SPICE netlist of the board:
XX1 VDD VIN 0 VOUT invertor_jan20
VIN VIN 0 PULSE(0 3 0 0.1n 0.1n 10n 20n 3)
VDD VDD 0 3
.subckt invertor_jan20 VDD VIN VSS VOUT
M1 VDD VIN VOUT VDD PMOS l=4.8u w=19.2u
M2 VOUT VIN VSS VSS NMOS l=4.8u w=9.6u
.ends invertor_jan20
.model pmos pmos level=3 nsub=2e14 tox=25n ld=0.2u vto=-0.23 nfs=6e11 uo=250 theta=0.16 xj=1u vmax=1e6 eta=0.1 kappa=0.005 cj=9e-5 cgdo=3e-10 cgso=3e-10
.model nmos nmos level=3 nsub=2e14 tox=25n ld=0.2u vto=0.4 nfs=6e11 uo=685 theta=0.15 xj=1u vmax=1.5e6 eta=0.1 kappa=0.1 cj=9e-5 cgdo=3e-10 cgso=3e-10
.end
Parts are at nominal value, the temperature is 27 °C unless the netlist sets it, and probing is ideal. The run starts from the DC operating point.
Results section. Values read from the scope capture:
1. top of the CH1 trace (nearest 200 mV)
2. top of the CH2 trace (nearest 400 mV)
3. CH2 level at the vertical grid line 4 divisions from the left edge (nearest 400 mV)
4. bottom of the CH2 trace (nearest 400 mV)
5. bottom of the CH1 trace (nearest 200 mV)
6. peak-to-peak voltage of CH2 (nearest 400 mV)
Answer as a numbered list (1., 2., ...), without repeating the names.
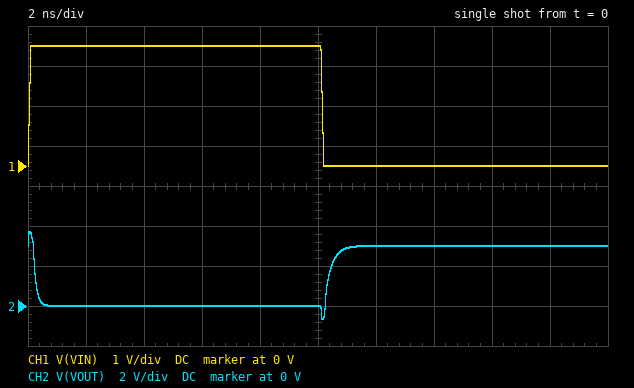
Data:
1. 3.0 V
2. 3.6 V
3. 0 V
4. -800 mV
5. 0 V
6. 4.4 V
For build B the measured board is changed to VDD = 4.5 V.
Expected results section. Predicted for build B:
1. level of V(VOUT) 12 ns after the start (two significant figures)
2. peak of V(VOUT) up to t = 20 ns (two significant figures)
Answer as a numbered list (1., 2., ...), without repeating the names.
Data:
1. 4.5 V
2. 5.2 V
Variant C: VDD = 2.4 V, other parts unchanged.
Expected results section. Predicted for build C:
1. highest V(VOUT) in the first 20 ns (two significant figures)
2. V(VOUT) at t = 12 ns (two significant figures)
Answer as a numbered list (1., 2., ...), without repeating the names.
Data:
1. 3.1 V
2. 2.4 V
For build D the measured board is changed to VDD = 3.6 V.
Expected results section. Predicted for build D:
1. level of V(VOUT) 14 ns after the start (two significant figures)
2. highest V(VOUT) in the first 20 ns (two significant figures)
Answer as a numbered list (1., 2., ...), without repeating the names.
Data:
1. 3.6 V
2. 4.3 V
